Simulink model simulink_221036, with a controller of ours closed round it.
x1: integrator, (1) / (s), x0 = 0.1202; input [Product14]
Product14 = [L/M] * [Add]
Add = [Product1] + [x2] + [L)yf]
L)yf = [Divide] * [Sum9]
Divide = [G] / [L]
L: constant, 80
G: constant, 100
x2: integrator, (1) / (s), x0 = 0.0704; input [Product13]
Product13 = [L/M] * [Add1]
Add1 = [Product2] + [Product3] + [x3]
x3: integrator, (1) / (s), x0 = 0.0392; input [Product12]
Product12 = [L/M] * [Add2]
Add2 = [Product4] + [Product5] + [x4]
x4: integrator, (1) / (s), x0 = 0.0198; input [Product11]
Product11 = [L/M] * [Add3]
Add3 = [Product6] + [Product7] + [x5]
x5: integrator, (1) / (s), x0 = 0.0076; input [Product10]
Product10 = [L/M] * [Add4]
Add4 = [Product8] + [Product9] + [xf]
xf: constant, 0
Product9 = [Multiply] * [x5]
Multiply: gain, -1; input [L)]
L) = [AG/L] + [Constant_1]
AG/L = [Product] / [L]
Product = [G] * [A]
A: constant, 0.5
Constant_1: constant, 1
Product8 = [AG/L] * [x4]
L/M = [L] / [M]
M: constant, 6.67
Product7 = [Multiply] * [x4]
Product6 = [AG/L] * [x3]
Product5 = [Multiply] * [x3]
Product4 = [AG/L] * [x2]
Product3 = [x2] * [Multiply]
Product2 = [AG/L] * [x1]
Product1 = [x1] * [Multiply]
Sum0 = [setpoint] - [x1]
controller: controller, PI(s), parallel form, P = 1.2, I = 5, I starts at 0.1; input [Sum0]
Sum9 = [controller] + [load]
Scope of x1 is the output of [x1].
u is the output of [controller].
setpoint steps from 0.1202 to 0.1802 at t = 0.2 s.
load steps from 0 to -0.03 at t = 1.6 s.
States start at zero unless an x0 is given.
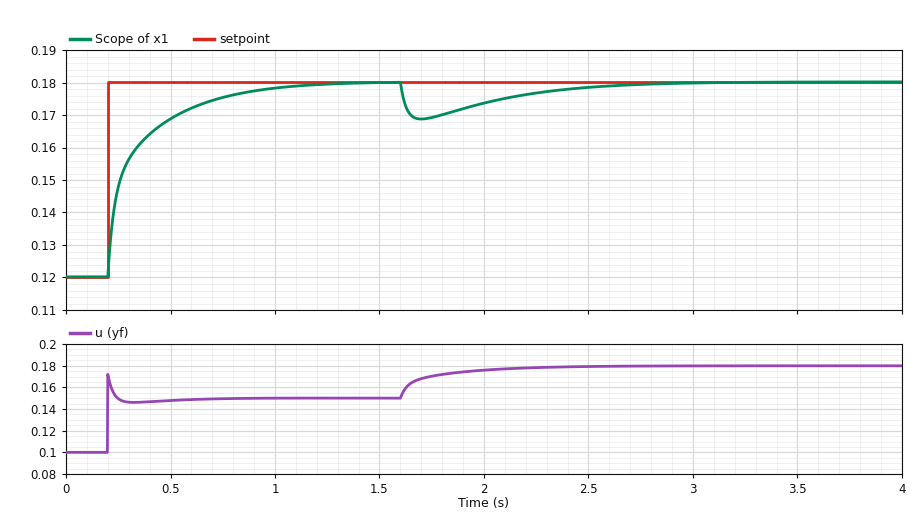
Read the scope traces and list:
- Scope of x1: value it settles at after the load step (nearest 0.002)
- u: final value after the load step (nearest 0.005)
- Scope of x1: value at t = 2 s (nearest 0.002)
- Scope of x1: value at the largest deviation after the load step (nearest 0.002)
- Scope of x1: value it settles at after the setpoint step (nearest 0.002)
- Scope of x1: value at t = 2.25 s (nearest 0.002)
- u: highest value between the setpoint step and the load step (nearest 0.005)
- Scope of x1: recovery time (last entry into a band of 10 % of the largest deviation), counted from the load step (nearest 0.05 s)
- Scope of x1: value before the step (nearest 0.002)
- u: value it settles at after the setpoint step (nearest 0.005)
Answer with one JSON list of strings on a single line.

["0.180", "0.180", "0.174", "0.168", "0.180", "0.176", "0.170", "1.05 s", "0.120", "0.150"]
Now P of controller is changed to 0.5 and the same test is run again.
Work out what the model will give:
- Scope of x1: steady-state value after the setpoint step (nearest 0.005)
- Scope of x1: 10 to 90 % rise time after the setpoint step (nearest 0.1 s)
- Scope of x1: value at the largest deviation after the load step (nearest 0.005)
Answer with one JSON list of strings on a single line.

["0.180", "0.4 s", "0.165"]
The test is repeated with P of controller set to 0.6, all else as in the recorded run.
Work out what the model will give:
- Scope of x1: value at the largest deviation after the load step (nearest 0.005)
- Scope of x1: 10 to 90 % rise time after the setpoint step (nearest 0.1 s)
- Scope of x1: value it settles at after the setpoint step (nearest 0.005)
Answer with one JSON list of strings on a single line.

["0.165", "0.4 s", "0.180"]
